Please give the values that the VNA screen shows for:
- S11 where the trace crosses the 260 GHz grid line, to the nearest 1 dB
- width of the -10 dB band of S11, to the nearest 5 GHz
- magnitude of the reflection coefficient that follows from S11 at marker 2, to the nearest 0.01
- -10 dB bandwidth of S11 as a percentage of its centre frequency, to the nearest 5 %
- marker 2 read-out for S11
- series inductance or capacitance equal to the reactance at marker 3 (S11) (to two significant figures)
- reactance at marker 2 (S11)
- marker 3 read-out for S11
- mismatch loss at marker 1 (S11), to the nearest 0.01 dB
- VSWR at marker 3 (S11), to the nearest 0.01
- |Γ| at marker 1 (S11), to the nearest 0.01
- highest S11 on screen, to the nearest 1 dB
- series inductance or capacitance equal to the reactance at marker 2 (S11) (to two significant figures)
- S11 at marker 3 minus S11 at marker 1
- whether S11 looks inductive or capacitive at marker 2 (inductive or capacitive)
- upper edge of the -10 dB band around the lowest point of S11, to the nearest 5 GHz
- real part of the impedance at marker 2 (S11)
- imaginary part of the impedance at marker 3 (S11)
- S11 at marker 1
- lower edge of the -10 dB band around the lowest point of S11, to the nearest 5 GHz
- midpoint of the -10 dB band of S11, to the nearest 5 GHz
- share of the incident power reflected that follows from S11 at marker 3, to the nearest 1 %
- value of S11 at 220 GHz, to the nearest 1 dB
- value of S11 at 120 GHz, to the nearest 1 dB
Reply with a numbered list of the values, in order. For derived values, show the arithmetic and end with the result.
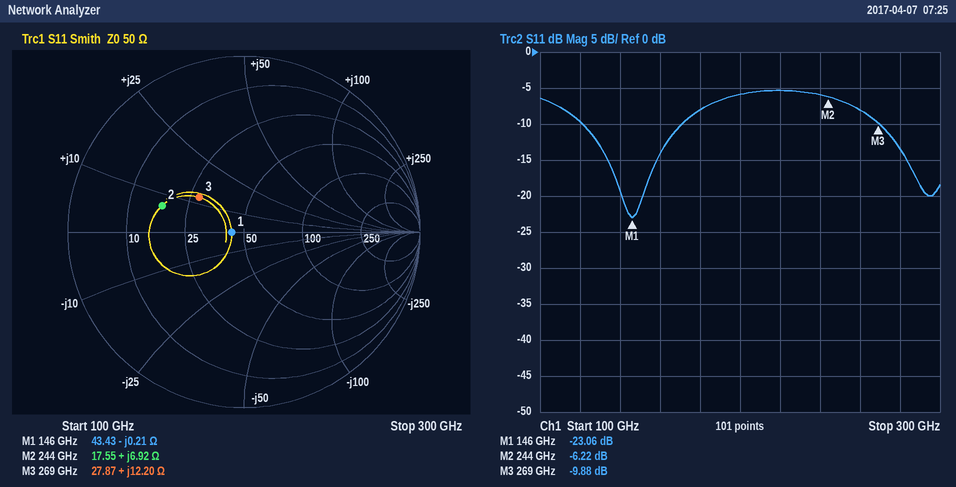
1. -8 dB
2. 170 GHz − 120 GHz = 50 GHz
3. 10^(-6.22/20) ≈ 0.49
4. 50 GHz / 145 GHz ≈ 35 %
5. -6.22 dB
6. L = 12.2 Ω/(2π × 269 GHz) ≈ 7.2 pH
7. +6.92 Ω
8. -9.88 dB
9. −10 log10(1 − 10^(-23.06/10)) ≈ 0.02 dB
10. 1.94
11. 0.07
12. -5 dB
13. L = 6.92 Ω/(2π × 244 GHz) ≈ 4.5 pH
14. -9.88 − (-23.06) = 13.18 dB
15. inductive
16. 170 GHz
17. 17.55 Ω
18. +12.20 Ω
19. -23.06 dB
20. 120 GHz
21. 145 GHz
22. 10^(-9.88/10) ≈ 10 %
23. -5 dB
24. -10 dB
